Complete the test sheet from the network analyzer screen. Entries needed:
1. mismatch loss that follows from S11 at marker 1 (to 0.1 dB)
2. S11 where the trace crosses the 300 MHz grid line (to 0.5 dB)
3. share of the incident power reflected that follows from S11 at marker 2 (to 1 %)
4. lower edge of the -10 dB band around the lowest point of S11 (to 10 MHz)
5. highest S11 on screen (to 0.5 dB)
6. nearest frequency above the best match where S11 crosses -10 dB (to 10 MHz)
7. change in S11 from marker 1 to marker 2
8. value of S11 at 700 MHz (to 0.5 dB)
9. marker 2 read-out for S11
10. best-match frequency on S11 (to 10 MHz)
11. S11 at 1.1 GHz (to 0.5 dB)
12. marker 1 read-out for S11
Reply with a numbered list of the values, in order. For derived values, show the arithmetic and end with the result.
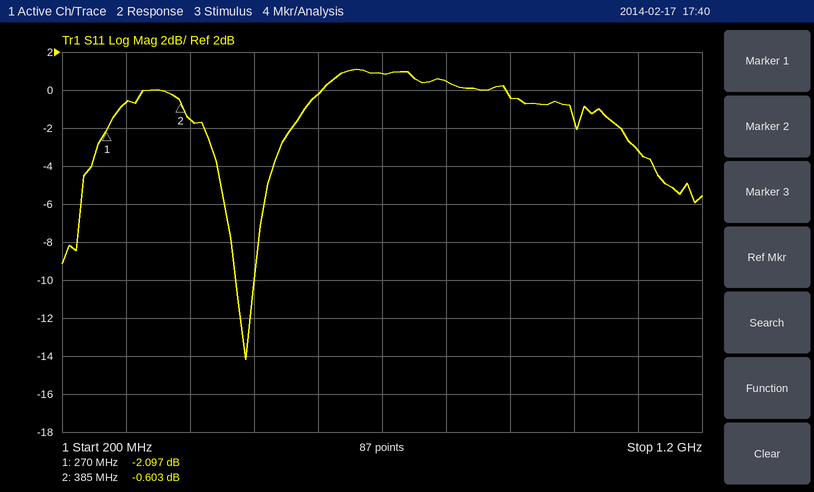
1. −10 log10(1 − 10^(-2.097/10)) ≈ 4.2 dB
2. -0.5 dB
3. 10^(-0.603/10) ≈ 87 %
4. 470 MHz
5. 1.0 dB
6. 500 MHz
7. -0.603 − (-2.097) = 1.494 dB
8. 1.0 dB
9. -0.603 dB
10. 490 MHz
11. -3.0 dB
12. -2.097 dB
